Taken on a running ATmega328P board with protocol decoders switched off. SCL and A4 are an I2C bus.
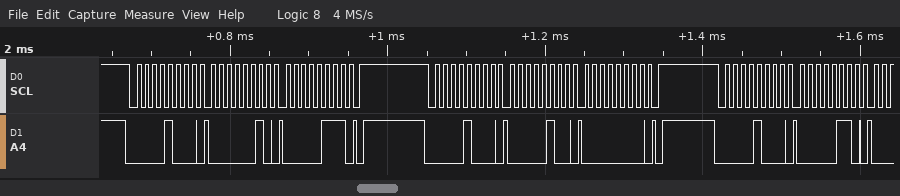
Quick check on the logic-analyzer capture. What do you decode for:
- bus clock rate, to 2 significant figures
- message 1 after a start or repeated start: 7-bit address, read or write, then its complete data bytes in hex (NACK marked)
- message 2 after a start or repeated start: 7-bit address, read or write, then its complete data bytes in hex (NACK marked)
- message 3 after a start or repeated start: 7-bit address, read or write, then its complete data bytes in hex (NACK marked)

100 kHz
0x04 write: 02 07
0x04 write: 04 00
0x04 write: 06
